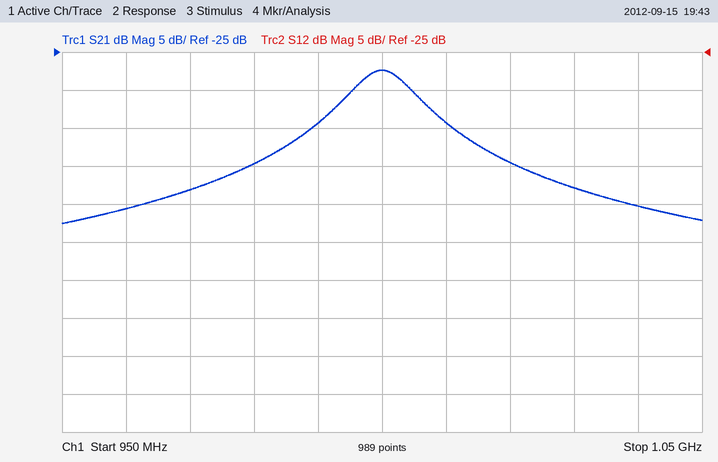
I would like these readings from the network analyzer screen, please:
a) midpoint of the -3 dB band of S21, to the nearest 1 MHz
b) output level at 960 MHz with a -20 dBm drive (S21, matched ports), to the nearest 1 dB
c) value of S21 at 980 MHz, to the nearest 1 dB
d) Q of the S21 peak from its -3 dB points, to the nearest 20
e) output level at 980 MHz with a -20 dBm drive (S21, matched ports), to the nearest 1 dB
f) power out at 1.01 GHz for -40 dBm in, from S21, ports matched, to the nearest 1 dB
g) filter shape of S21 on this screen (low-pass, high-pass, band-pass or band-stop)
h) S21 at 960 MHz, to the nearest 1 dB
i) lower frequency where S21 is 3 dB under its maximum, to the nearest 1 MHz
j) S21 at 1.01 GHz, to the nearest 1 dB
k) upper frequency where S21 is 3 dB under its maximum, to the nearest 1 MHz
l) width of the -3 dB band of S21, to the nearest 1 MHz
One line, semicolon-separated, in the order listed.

1.000 GHz; -66 dBm; -40 dB; 100; -60 dBm; -74 dBm; band-pass; -46 dB; 995 MHz; -34 dB; 1.005 GHz; 10 MHz
